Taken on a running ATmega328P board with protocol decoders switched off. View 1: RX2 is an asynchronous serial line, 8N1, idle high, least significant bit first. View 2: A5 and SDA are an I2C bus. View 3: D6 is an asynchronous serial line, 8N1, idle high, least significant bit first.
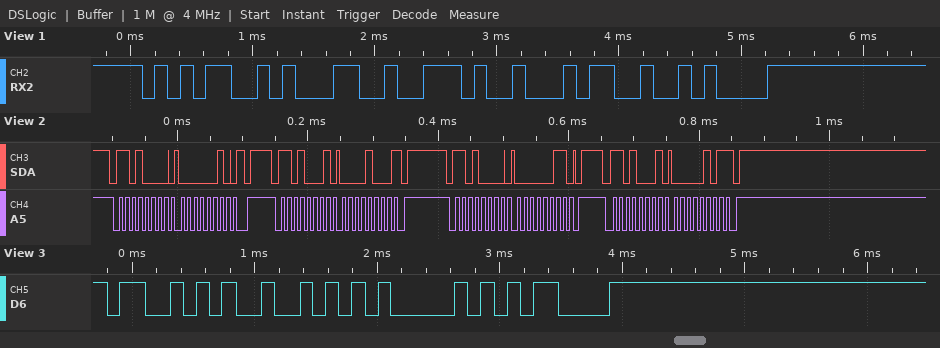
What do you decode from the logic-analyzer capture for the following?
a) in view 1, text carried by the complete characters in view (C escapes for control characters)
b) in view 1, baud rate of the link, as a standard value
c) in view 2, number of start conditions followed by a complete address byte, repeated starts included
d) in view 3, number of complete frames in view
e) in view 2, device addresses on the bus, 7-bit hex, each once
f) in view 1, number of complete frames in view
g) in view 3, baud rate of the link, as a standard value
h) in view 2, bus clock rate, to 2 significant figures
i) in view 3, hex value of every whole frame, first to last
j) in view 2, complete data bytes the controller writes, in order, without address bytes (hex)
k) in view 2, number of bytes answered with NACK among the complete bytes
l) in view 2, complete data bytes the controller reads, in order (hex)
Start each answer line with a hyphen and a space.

- "51.4\n"
- 9600 baud
- 4
- 4
- 0x68
- 5
- 9600 baud
- 100 kHz
- 53 52 41 0D
- 02 03
- 2
- 08 05
